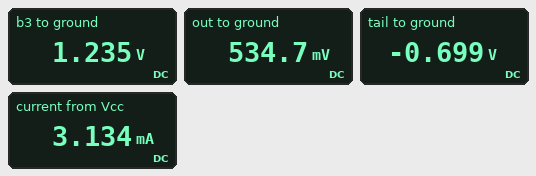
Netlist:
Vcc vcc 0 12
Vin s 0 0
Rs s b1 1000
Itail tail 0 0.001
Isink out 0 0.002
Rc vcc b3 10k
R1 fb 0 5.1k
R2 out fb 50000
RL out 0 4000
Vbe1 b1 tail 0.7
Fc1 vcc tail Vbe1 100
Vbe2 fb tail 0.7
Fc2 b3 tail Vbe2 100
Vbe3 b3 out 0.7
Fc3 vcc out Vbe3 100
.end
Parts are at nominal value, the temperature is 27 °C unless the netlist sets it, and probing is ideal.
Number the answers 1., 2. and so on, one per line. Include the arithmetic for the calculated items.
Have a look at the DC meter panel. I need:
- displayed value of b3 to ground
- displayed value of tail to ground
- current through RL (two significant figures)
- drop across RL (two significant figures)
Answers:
1. 1.235 V
2. -0.699 V
3. (534.7 mV) / 4 kΩ = 130 µA
4. 534.7 mV = 530 mV
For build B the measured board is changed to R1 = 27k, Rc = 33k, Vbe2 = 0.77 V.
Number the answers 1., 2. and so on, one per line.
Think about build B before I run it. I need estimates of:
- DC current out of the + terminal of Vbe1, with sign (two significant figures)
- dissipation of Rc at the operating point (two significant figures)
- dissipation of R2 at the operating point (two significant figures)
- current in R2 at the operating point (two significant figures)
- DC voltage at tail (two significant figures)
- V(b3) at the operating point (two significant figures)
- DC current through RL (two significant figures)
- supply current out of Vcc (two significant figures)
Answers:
1. -6.8 µA
2. 3.6 mW
3. 1.5 µW
4. 5.5 µA
5. -710 mV
6. 1.0 V
7. 84 µA
8. 3.1 mA
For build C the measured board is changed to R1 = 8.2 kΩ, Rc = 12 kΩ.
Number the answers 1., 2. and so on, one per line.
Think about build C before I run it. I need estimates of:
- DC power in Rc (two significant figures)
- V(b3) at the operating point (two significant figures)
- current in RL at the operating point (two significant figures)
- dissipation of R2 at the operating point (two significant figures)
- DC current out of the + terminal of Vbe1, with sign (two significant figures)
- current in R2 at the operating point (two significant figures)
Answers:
1. 9.8 mW
2. 1.1 V
3. 110 µA
4. 3.8 µW
5. -1.1 µA
6. 8.7 µA
